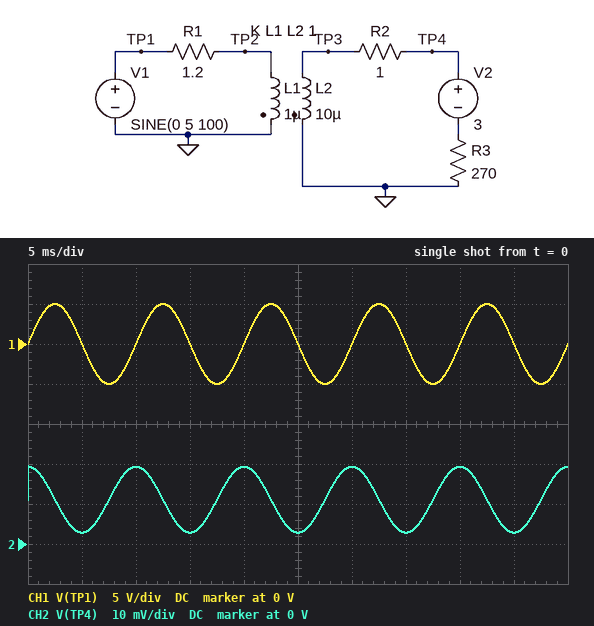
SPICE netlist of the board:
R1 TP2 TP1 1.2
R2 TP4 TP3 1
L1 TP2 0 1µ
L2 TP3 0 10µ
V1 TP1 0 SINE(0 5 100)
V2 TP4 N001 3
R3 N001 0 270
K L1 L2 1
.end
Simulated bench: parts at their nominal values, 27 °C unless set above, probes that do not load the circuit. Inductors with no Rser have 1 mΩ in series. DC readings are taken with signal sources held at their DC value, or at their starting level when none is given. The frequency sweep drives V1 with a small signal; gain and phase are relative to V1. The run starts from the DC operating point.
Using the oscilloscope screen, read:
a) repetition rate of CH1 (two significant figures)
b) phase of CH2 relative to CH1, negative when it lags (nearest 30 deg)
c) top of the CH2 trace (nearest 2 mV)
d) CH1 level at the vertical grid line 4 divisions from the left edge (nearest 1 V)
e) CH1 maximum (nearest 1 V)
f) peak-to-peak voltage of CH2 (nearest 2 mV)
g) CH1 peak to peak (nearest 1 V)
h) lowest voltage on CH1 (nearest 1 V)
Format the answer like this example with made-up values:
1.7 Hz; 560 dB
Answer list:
100 Hz; 90 deg; 20 mV; 0 V; 5 V; 16 mV; 10 V; -5 V
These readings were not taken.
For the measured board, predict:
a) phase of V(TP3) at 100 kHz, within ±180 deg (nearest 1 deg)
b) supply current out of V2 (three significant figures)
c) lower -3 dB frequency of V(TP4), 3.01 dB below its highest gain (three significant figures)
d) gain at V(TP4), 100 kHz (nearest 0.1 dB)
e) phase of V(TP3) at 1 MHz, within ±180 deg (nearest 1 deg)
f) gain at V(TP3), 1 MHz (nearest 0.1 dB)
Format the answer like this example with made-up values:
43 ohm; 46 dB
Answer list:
61 deg; 11.1 mA; 183 kHz; 3.2 dB; 10 deg; 9.5 dB
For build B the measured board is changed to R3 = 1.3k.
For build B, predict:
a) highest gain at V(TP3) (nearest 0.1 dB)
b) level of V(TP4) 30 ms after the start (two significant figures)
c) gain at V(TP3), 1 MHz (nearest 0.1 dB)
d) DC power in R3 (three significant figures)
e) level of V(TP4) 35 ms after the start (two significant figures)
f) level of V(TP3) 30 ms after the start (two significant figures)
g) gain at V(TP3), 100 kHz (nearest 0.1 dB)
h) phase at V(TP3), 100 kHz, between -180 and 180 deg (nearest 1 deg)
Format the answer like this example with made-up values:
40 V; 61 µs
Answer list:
9.9 dB; 11 mV; 9.8 dB; 6.91 mW; -6.0 mV; 8.3 mV; 3.3 dB; 62 deg
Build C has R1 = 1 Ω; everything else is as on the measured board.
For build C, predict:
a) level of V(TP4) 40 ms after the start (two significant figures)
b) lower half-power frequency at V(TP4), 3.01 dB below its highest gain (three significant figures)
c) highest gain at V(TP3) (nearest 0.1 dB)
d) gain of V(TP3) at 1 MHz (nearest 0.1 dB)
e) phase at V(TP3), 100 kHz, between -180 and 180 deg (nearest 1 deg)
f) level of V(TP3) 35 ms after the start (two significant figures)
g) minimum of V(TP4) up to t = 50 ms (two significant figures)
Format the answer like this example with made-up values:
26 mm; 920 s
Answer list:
21 mV; 154 kHz; 9.7 dB; 9.6 dB; 57 deg; -9.9 mV; 1.2 mV
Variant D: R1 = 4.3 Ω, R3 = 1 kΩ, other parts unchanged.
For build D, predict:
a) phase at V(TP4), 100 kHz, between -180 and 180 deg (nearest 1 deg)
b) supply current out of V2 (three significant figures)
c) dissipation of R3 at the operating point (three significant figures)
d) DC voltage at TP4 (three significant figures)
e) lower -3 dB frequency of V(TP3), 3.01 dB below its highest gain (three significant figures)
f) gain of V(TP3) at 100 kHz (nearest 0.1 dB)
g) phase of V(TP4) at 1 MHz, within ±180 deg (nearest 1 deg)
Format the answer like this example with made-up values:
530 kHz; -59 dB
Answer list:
81 deg; 3.00 mA; 8.98 mW; 3.00 mV; 656 kHz; -6.8 dB; 33 deg
